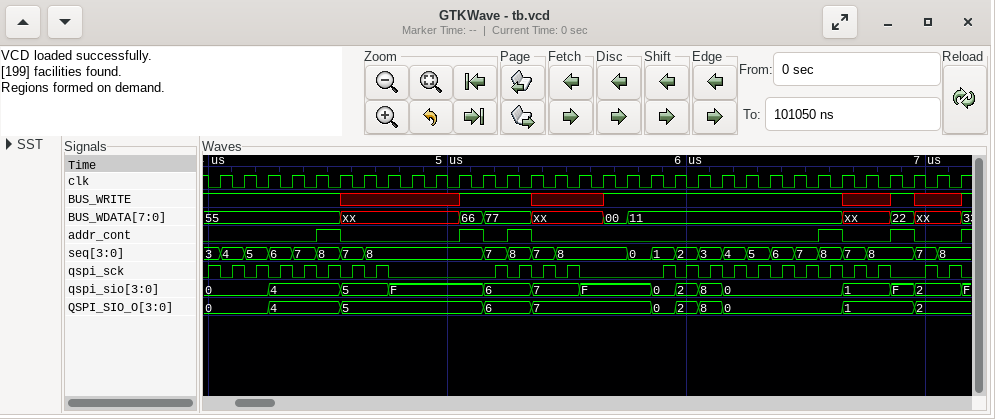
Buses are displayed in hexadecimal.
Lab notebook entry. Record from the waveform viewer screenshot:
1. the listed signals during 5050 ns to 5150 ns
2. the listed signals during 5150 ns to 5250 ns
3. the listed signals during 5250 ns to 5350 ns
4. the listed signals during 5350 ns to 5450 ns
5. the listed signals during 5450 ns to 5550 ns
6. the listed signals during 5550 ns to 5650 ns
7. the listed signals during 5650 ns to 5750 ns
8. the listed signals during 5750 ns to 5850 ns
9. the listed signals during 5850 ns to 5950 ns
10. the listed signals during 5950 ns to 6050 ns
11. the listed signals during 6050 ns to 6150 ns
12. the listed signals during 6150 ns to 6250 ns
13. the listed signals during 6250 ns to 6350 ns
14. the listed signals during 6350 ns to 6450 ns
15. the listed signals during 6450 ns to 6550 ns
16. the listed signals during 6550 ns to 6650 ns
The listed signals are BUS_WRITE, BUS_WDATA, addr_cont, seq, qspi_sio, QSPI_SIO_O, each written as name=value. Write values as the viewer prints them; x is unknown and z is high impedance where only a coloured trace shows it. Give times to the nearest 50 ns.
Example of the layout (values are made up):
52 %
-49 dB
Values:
BUS_WRITE=1, BUS_WDATA=66, addr_cont=1, seq=8, qspi_sio=F, QSPI_SIO_O=5
BUS_WRITE=1, BUS_WDATA=77, addr_cont=0, seq=7, qspi_sio=6, QSPI_SIO_O=6
BUS_WRITE=1, BUS_WDATA=77, addr_cont=1, seq=8, qspi_sio=6, QSPI_SIO_O=6
BUS_WRITE=x, BUS_WDATA=xx, addr_cont=0, seq=7, qspi_sio=7, QSPI_SIO_O=7
BUS_WRITE=x, BUS_WDATA=xx, addr_cont=0, seq=8, qspi_sio=7, QSPI_SIO_O=7
BUS_WRITE=x, BUS_WDATA=xx, addr_cont=0, seq=8, qspi_sio=F, QSPI_SIO_O=7
BUS_WRITE=1, BUS_WDATA=00, addr_cont=0, seq=8, qspi_sio=F, QSPI_SIO_O=7
BUS_WRITE=1, BUS_WDATA=11, addr_cont=0, seq=0, qspi_sio=F, QSPI_SIO_O=7
BUS_WRITE=1, BUS_WDATA=11, addr_cont=0, seq=1, qspi_sio=0, QSPI_SIO_O=0
BUS_WRITE=1, BUS_WDATA=11, addr_cont=0, seq=2, qspi_sio=2, QSPI_SIO_O=2
BUS_WRITE=1, BUS_WDATA=11, addr_cont=0, seq=3, qspi_sio=8, QSPI_SIO_O=8
BUS_WRITE=1, BUS_WDATA=11, addr_cont=0, seq=4, qspi_sio=0, QSPI_SIO_O=0
BUS_WRITE=1, BUS_WDATA=11, addr_cont=0, seq=5, qspi_sio=0, QSPI_SIO_O=0
BUS_WRITE=1, BUS_WDATA=11, addr_cont=0, seq=6, qspi_sio=0, QSPI_SIO_O=0
BUS_WRITE=1, BUS_WDATA=11, addr_cont=0, seq=7, qspi_sio=0, QSPI_SIO_O=0
BUS_WRITE=1, BUS_WDATA=11, addr_cont=1, seq=8, qspi_sio=0, QSPI_SIO_O=0
